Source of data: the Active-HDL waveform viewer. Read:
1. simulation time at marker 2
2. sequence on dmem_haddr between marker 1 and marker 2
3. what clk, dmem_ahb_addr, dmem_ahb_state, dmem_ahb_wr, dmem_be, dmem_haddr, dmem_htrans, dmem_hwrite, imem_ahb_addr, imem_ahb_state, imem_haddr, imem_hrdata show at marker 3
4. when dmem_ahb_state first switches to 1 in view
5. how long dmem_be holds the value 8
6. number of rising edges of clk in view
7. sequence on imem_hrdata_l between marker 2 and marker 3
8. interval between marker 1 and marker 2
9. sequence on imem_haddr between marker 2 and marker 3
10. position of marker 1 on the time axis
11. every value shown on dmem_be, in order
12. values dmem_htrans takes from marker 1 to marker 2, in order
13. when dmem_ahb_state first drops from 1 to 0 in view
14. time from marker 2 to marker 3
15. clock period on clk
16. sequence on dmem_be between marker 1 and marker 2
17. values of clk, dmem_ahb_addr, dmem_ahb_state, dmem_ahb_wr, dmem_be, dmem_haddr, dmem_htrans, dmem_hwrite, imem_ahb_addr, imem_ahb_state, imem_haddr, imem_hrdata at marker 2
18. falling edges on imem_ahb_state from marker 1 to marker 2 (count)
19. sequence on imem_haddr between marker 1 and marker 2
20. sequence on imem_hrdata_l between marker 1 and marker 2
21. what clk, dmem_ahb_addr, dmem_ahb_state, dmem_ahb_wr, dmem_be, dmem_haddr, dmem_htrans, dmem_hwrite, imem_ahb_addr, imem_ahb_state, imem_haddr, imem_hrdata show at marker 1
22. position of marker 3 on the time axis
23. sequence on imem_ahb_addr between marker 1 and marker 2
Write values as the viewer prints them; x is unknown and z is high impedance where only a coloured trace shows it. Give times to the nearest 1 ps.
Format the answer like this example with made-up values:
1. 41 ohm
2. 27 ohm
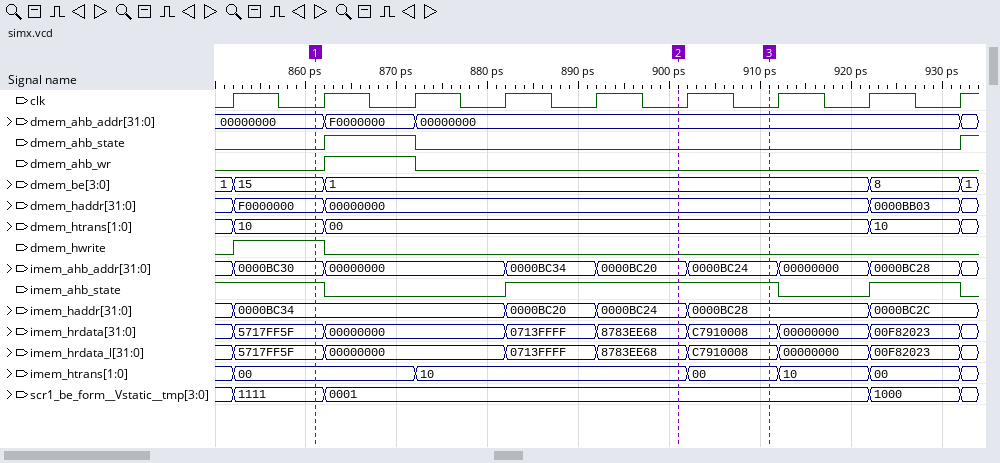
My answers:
1. 901 ps
2. F0000000, 00000000
3. clk=0, dmem_ahb_addr=00000000, dmem_ahb_state=0, dmem_ahb_wr=0, dmem_be=1, dmem_haddr=00000000, dmem_htrans=00, dmem_hwrite=0, imem_ahb_addr=0000BC24, imem_ahb_state=1, imem_haddr=0000BC28, imem_hrdata=C7910008
4. 862 ps
5. 10 ps
6. 9
7. 8783EE68, C7910008
8. 40 ps
9. 0000BC24, 0000BC28
10. 861 ps
11. 1, 15, 1, 8, 1
12. 10, 00
13. 872 ps
14. 10 ps
15. 10 ps
16. 15, 1
17. clk=0, dmem_ahb_addr=00000000, dmem_ahb_state=0, dmem_ahb_wr=0, dmem_be=1, dmem_haddr=00000000, dmem_htrans=00, dmem_hwrite=0, imem_ahb_addr=0000BC20, imem_ahb_state=1, imem_haddr=0000BC24, imem_hrdata=8783EE68
18. 1
19. 0000BC34, 0000BC20, 0000BC24
20. 5717FF5F, 00000000, 0713FFFF, 8783EE68
21. clk=0, dmem_ahb_addr=00000000, dmem_ahb_state=0, dmem_ahb_wr=0, dmem_be=15, dmem_haddr=F0000000, dmem_htrans=10, dmem_hwrite=1, imem_ahb_addr=0000BC30, imem_ahb_state=1, imem_haddr=0000BC34, imem_hrdata=5717FF5F
22. 911 ps
23. 0000BC30, 00000000, 0000BC34, 0000BC20
